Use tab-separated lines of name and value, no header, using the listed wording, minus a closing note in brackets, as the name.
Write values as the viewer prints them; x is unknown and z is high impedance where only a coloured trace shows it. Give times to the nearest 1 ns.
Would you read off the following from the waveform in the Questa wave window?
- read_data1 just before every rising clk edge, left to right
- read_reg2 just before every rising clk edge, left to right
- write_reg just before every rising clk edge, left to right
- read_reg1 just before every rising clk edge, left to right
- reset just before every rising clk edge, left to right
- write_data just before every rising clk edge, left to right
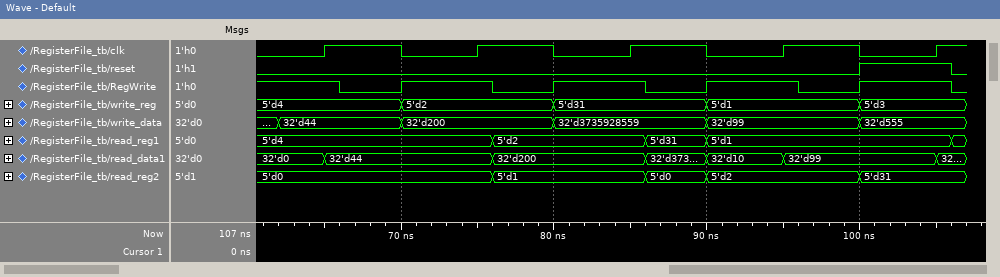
read_data1 just before every rising clk edge, left to right	32'd0, 32'd44, 32'd200, 32'd10, 32'd99
read_reg2 just before every rising clk edge, left to right	5'd0, 5'd0, 5'd1, 5'd2, 5'd31
write_reg just before every rising clk edge, left to right	5'd4, 5'd2, 5'd31, 5'd1, 5'd3
read_reg1 just before every rising clk edge, left to right	5'd4, 5'd4, 5'd2, 5'd1, 5'd1
reset just before every rising clk edge, left to right	0 0 0 0 1
write_data just before every rising clk edge, left to right	32'd44, 32'd200, 32'd3735928559, 32'd99, 32'd555
